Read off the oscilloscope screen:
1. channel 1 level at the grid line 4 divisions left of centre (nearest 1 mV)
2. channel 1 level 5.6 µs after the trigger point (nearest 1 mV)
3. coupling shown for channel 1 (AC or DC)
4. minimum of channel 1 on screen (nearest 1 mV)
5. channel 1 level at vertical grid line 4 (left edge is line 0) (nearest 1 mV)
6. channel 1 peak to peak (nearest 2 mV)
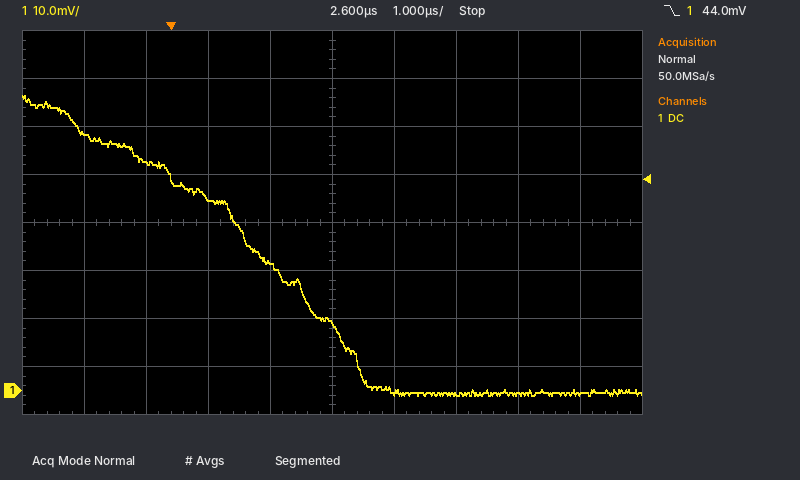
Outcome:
54 mV
-1 mV
DC
-1 mV
27 mV
62 mV
